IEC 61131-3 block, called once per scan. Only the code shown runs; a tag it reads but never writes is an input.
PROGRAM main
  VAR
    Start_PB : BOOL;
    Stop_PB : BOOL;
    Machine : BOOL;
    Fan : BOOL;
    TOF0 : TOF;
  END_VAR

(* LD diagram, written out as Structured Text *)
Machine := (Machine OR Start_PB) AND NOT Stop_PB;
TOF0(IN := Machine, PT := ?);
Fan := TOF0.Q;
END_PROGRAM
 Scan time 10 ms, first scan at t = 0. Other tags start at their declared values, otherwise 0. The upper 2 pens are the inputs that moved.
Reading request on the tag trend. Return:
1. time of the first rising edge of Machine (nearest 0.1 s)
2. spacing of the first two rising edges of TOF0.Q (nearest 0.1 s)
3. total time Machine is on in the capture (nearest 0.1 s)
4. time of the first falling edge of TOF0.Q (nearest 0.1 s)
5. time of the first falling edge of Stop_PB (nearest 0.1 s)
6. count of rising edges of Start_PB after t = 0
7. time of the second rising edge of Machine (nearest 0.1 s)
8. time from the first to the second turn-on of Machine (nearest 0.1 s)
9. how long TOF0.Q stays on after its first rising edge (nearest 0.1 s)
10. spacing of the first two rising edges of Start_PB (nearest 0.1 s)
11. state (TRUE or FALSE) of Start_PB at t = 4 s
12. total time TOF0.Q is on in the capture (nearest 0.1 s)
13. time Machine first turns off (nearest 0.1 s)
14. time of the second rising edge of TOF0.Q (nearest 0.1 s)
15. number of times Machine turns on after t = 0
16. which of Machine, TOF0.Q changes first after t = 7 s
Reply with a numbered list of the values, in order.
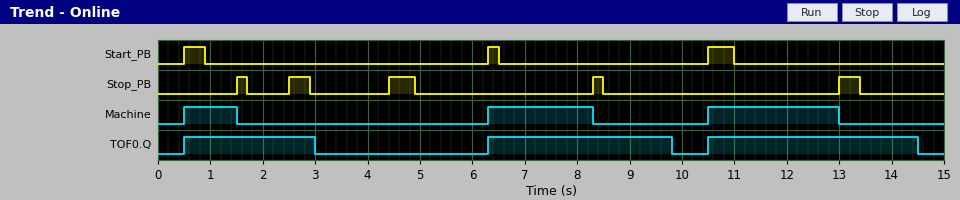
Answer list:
1. 0.5 s
2. 5.8 s
3. 5.5 s
4. 3.0 s
5. 1.7 s
6. 3
7. 6.3 s
8. 5.8 s
9. 2.5 s
10. 5.8 s
11. FALSE
12. 10.0 s
13. 1.5 s
14. 6.3 s
15. 3
16. Machine
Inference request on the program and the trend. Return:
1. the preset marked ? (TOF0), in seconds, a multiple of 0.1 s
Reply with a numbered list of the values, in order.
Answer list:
1. 1.5 s
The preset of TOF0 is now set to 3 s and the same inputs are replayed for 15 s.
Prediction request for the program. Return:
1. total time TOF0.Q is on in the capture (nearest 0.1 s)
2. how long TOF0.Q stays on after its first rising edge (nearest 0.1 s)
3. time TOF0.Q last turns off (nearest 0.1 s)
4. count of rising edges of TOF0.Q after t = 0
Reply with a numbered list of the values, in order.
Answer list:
1. 12.7 s
2. 4.0 s
3. 4.5 s
4. 2
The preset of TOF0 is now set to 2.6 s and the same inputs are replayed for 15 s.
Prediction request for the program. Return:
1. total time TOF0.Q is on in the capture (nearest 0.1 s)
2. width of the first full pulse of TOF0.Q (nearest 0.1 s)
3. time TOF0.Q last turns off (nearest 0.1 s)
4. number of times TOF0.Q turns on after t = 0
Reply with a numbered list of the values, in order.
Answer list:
1. 12.3 s
2. 3.6 s
3. 4.1 s
4. 2
